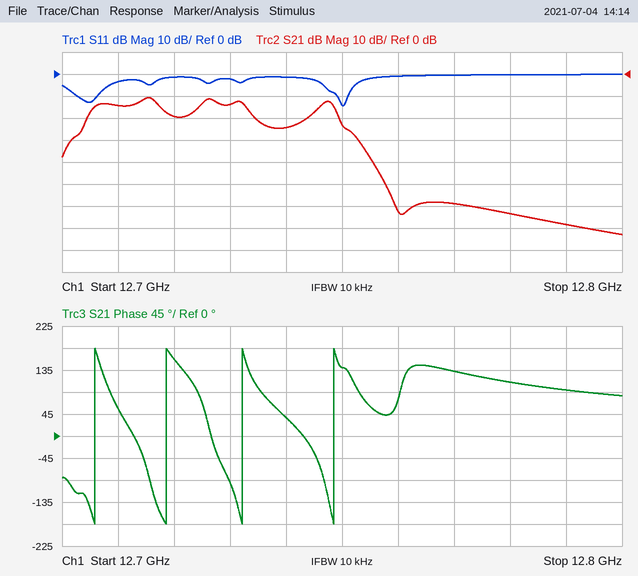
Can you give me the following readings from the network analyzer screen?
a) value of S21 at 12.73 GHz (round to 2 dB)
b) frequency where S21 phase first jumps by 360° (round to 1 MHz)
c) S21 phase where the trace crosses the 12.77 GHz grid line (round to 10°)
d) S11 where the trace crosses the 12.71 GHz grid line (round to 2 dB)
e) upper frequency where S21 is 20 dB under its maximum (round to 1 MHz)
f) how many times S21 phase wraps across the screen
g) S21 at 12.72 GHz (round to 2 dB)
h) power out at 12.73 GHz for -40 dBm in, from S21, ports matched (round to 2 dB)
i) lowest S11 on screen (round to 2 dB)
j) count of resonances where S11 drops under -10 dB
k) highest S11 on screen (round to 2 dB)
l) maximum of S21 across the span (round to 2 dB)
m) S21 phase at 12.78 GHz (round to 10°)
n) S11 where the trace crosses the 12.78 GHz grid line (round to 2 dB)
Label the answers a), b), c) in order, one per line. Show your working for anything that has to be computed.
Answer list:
a) -14 dB
b) 12.706 GHz
c) 130°
d) -4 dB
e) 12.753 GHz
f) 4
g) -20 dB
h) -40 dBm + (-14 dB) = -54 dBm
i) -14 dB
j) 2
k) 0 dB
l) -10 dB
m) 110°
n) 0 dB
